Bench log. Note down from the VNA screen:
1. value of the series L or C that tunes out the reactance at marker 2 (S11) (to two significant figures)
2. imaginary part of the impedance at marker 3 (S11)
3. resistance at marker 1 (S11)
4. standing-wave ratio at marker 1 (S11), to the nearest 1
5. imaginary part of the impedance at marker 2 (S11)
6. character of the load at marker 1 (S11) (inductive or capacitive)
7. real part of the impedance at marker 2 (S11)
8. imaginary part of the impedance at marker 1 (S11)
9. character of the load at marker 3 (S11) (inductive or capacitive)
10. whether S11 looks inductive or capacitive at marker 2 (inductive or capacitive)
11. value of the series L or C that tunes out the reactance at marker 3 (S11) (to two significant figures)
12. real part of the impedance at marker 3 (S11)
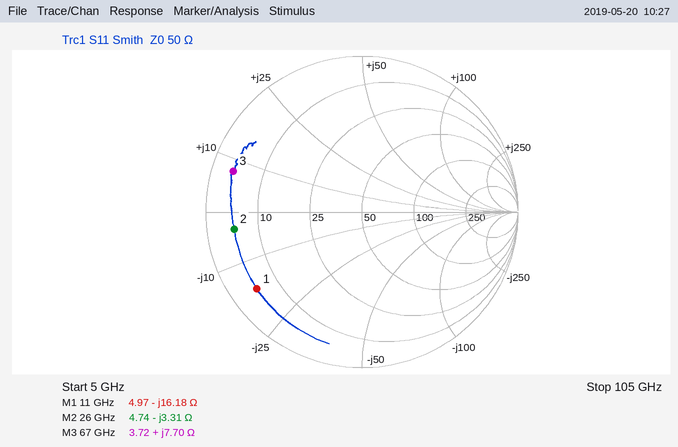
20 pH
+7.70 Ω
4.97 Ω
11
-3.31 Ω
capacitive
4.74 Ω
-16.18 Ω
inductive
capacitive
310 fF
3.72 Ω
